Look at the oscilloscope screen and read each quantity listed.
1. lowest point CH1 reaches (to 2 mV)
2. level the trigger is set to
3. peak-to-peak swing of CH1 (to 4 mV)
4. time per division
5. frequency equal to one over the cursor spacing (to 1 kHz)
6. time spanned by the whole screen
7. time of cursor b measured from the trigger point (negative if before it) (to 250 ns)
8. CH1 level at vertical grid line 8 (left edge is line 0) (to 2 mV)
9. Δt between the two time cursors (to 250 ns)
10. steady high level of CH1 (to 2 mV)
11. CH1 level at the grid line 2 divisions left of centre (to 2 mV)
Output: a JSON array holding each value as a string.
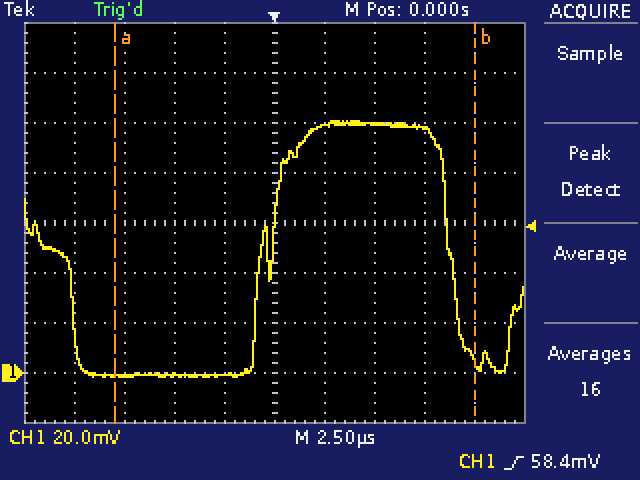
["-2 mV", "58.4 mV", "104 mV", "2.5 µs", "56 kHz", "25 µs", "+10.00 µs", "98 mV", "18.00 µs", "100 mV", "0 mV"]
